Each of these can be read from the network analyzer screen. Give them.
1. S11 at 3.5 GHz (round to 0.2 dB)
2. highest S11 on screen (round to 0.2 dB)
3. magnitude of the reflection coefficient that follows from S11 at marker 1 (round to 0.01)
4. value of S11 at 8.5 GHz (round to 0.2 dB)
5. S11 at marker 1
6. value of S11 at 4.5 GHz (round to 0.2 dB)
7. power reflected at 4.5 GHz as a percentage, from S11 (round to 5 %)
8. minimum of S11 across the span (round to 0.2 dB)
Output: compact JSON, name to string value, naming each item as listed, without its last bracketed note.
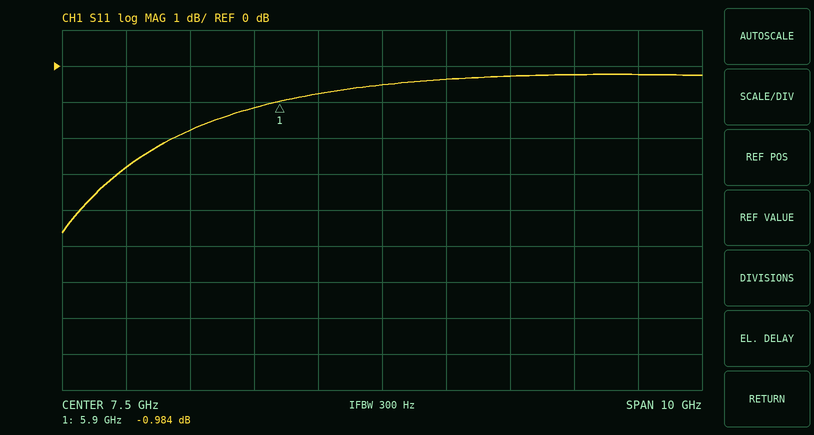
{"S11 at 3.5 GHz": "-2.8 dB", "highest S11 on screen": "-0.2 dB", "magnitude of the reflection coefficient that follows from S11 at marker 1": "0.89", "value of S11 at 8.5 GHz": "-0.4 dB", "S11 at marker 1": "-0.984 dB", "value of S11 at 4.5 GHz": "-1.8 dB", "power reflected at 4.5 GHz as a percentage, from S11": "65 %", "minimum of S11 across the span": "-4.6 dB"}
